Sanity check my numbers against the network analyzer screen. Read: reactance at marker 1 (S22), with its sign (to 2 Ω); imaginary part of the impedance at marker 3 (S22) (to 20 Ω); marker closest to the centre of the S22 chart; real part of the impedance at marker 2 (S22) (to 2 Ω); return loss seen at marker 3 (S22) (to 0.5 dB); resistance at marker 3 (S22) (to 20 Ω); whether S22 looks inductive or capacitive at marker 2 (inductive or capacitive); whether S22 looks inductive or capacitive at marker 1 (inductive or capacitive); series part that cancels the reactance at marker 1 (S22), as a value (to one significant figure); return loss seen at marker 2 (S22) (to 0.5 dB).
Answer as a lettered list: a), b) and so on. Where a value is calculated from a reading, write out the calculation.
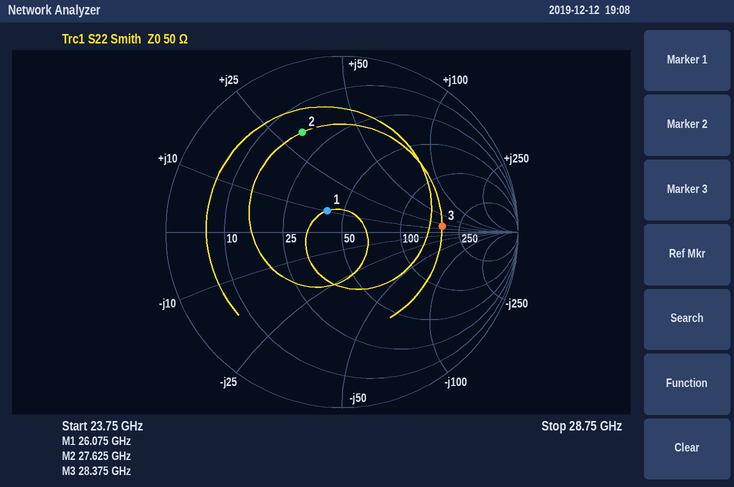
a) +10 Ω
b) +20 Ω
c) marker 1
d) 18 Ω
e) 5.0 dB
f) 180 Ω
g) inductive
h) inductive
i) C = 1/(2π × 26.075 GHz × 10 Ω) ≈ 610 fF, so 600 fF to one significant figure
j) 4.5 dB
